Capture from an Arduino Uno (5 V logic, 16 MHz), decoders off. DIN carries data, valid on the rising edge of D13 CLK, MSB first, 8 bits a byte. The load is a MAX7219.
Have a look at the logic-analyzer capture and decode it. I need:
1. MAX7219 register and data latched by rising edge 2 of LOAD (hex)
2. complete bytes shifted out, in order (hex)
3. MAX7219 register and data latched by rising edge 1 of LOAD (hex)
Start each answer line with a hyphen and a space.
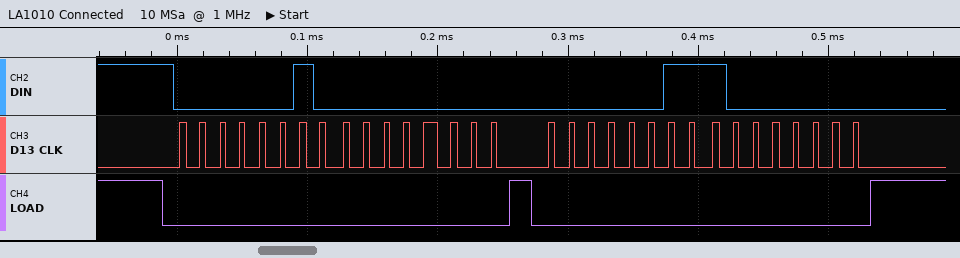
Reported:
- register 0x3, data 0x80
- 0x02 0x00 0x03 0x80
- register 0x2, data 0x00
